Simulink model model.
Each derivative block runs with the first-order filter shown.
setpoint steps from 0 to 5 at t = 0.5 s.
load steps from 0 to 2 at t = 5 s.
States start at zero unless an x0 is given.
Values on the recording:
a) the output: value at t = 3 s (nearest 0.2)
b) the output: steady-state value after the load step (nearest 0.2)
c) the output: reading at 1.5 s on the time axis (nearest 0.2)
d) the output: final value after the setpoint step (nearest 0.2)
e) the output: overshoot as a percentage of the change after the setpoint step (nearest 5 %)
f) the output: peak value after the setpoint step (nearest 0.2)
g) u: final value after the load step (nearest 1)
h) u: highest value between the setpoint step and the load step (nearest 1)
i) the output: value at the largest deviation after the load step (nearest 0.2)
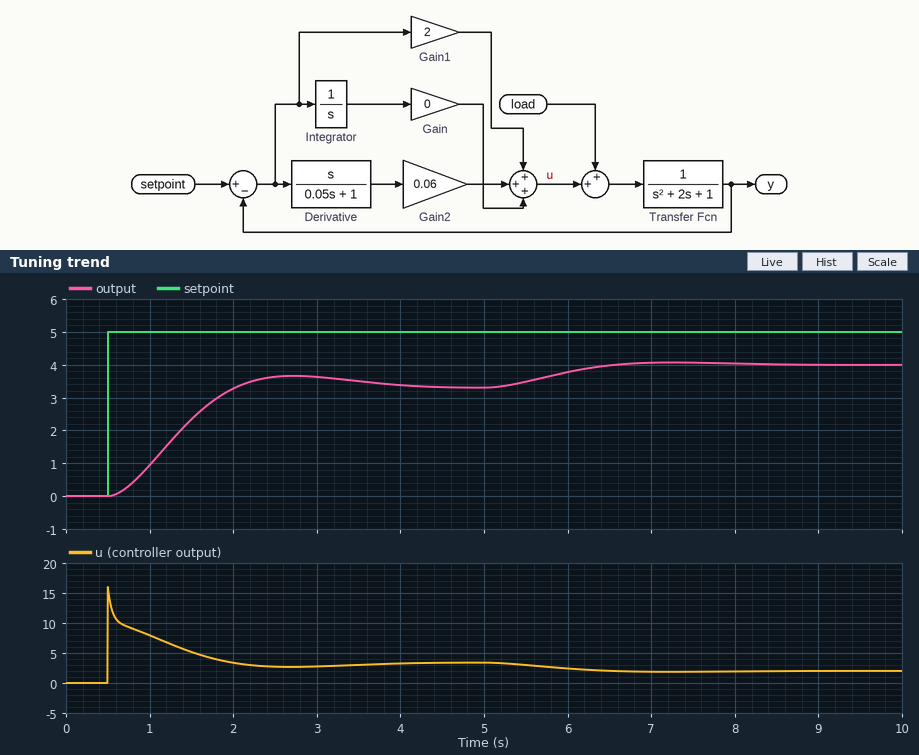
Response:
3.6
4.0
2.4
3.4
10 %
3.6
2
16
4.0
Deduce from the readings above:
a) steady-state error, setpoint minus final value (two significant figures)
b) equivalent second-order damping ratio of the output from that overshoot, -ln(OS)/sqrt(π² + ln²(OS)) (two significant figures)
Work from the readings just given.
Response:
1.6
0.59
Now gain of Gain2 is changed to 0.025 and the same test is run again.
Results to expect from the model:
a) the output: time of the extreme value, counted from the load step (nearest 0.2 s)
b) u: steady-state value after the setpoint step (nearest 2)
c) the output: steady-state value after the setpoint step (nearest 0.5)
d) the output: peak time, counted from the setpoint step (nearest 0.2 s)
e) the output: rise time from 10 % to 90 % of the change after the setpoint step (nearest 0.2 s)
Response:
2.2 s
4
3.5
2.2 s
1.0 s
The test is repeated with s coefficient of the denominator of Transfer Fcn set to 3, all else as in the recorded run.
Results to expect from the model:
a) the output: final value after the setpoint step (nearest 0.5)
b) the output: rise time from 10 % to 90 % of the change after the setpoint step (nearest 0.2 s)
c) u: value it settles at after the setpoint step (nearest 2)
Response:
3.5
1.6 s
4
